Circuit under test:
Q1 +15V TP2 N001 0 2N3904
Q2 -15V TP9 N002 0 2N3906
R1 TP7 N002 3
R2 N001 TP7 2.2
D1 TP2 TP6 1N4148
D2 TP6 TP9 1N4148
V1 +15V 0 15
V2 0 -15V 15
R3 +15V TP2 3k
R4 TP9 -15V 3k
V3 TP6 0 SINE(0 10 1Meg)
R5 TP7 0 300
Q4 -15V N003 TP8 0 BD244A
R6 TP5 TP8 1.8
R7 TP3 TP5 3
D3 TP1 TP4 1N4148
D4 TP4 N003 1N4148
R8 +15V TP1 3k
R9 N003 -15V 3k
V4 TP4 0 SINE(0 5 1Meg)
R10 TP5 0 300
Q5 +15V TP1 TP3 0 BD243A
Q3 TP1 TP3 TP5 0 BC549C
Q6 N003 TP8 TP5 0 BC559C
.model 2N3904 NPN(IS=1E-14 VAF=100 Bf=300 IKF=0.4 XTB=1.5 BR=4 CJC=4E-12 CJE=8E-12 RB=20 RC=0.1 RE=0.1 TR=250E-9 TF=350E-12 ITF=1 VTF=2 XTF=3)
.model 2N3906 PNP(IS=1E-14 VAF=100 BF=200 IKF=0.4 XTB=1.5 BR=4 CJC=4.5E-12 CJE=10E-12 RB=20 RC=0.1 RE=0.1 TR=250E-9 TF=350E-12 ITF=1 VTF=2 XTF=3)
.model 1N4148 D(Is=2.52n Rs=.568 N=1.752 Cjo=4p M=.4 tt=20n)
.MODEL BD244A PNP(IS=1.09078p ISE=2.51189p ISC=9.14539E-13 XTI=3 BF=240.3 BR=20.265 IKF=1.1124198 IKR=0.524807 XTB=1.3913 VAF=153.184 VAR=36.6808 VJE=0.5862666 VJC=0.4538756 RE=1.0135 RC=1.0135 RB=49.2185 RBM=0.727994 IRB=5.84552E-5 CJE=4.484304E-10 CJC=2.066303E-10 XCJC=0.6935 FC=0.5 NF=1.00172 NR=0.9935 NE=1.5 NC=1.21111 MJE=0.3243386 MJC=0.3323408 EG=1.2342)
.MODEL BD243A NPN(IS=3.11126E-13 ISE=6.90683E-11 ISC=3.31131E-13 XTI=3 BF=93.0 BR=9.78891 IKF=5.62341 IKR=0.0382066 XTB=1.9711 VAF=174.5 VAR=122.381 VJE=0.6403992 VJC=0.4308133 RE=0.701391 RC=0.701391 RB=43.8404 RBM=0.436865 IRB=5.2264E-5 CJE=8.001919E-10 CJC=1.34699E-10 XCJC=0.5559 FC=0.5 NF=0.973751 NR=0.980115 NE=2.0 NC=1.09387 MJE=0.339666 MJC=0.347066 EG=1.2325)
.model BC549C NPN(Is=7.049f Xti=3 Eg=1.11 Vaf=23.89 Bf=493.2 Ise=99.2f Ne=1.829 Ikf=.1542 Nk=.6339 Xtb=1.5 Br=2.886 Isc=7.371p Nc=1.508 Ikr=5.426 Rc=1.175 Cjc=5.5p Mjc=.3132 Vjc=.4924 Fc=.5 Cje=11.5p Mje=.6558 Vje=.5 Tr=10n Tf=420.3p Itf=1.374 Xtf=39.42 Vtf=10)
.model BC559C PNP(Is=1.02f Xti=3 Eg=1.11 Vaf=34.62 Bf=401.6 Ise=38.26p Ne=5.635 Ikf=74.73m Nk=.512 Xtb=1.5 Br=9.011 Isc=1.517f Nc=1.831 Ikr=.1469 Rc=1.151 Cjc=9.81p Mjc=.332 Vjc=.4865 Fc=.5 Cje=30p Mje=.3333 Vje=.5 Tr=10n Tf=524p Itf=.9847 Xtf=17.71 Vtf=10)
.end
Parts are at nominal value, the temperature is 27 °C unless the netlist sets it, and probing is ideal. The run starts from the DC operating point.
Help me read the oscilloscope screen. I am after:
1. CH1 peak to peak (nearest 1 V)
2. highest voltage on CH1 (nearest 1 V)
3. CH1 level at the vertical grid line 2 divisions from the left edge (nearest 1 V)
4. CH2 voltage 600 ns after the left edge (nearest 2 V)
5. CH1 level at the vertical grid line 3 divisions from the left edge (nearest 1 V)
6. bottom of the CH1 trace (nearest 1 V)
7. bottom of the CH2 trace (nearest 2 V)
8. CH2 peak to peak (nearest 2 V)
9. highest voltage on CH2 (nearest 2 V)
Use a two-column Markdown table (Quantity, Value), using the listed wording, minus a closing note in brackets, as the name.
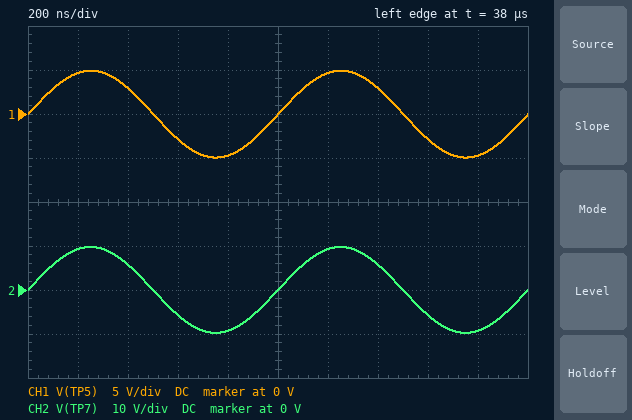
| Quantity | Value |
|---|---|
| CH1 peak to peak | 10 V |
| highest voltage on CH1 | 5 V |
| CH1 level at the vertical grid line 2 divisions from the left edge | 3 V |
| CH2 voltage 600 ns after the left edge | -6 V |
| CH1 level at the vertical grid line 3 divisions from the left edge | -3 V |
| bottom of the CH1 trace | -5 V |
| bottom of the CH2 trace | -10 V |
| CH2 peak to peak | 20 V |
| highest voltage on CH2 | 10 V |
